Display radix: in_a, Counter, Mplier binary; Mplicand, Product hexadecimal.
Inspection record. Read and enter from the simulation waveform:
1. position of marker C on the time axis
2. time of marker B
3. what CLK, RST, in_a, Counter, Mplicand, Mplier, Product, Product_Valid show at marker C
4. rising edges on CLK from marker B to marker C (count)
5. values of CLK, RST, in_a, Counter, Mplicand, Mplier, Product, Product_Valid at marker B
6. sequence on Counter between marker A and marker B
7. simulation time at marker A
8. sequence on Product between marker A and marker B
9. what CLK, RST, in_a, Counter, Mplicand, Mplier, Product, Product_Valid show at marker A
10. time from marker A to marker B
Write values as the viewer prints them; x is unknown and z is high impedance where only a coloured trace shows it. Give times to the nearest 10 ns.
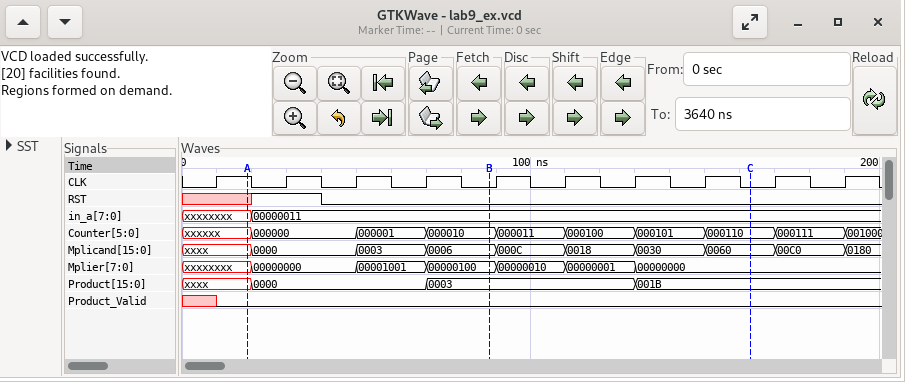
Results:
160 ns
90 ns
CLK=0, RST=0, in_a=00000011, Counter=000110, Mplicand=0060, Mplier=00000000, Product=001B, Product_Valid=0
4
CLK=0, RST=0, in_a=00000011, Counter=000010, Mplicand=0006, Mplier=00000100, Product=0003, Product_Valid=0
xxxxxx, 000000, 000001, 000010
20 ns
xxxx, 0000, 0003
CLK=1, RST=x, in_a=xxxxxxxx, Counter=xxxxxx, Mplicand=xxxx, Mplier=xxxxxxxx, Product=xxxx, Product_Valid=0
70 ns
